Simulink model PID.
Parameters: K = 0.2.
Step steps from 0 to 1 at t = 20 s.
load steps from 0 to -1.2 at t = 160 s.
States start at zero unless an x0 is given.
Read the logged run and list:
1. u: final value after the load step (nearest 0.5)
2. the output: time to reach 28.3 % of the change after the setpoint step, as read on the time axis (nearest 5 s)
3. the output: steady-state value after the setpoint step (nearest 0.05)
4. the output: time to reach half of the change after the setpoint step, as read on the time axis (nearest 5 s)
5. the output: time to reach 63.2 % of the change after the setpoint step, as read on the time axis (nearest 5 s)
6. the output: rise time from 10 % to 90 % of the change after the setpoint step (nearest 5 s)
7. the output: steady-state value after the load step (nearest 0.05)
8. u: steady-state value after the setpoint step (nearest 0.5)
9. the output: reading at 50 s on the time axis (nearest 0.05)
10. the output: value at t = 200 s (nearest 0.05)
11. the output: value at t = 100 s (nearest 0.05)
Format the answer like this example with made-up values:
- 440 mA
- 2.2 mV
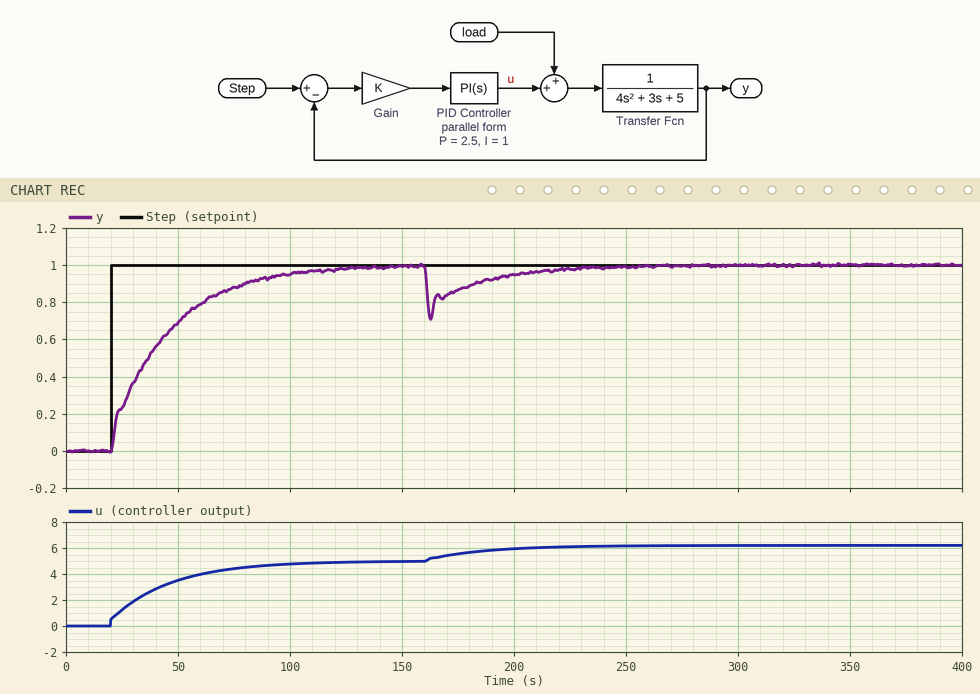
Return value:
- 6.0
- 25 s
- 1.00
- 35 s
- 45 s
- 60 s
- 1.00
- 5.0
- 0.70
- 0.95
- 0.95
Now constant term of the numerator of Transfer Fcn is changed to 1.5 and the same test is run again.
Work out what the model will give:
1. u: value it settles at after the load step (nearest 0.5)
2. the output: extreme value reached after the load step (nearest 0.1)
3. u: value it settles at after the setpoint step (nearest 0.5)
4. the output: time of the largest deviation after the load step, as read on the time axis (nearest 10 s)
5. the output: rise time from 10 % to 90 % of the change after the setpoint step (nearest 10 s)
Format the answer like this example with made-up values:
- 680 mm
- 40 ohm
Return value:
- 4.5
- 0.6
- 3.5
- 160 s
- 40 s
